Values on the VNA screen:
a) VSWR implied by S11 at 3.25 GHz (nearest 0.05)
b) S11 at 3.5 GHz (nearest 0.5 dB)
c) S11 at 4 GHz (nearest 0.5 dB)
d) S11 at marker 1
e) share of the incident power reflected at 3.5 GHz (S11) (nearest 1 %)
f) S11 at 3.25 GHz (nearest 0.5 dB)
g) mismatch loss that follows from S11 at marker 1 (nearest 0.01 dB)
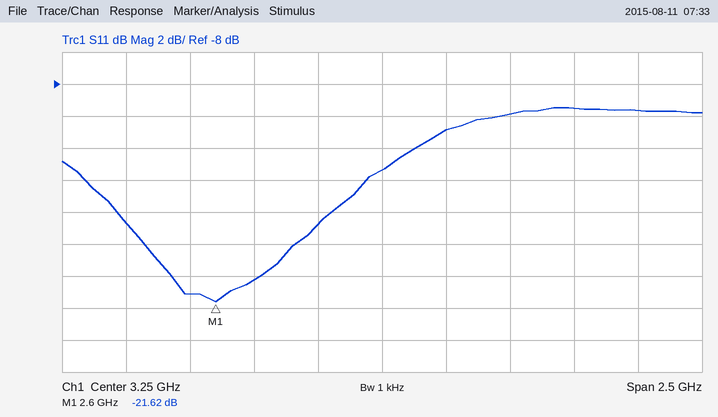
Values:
1.55
-11.0 dB
-9.5 dB
-21.62 dB
8 %
-13.5 dB
0.03 dB
